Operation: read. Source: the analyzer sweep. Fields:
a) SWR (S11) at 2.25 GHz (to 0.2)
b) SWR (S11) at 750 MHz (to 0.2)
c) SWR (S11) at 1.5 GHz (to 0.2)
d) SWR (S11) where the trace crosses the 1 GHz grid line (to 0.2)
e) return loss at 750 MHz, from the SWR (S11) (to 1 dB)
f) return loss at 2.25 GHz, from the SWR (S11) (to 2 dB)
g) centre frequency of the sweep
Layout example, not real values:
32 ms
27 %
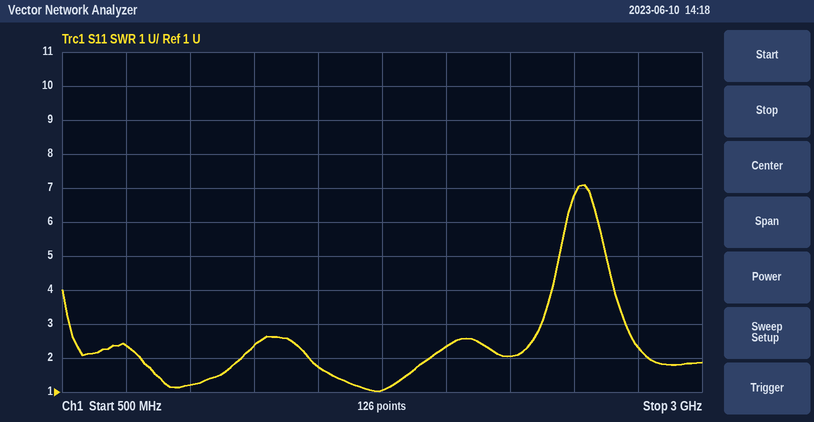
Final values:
2.0
2.4
1.8
1.2
8 dB
10 dB
1.75 GHz
